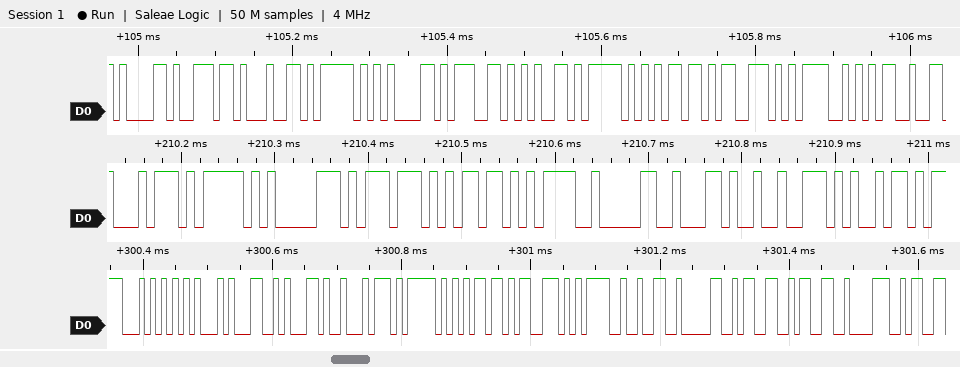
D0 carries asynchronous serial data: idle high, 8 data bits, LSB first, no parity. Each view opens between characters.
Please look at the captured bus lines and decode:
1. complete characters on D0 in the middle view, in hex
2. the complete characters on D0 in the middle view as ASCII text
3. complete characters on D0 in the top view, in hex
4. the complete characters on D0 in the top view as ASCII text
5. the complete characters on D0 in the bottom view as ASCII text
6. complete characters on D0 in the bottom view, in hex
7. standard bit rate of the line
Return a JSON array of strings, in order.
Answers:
["74, 5F, 70, 77, 6D, 3D, 30, 2C, 72, 69", "\"t_pwm=0,ri\"", "61, 6E, 64, 5F, 61, 67, 65, 5F, 6D, 73, 3D, 35", "\"and_age_ms=5\"", "\"TEL,t_ms=20338\"", "54, 45, 4C, 2C, 74, 5F, 6D, 73, 3D, 32, 30, 33, 33, 38", "115200 baud"]
